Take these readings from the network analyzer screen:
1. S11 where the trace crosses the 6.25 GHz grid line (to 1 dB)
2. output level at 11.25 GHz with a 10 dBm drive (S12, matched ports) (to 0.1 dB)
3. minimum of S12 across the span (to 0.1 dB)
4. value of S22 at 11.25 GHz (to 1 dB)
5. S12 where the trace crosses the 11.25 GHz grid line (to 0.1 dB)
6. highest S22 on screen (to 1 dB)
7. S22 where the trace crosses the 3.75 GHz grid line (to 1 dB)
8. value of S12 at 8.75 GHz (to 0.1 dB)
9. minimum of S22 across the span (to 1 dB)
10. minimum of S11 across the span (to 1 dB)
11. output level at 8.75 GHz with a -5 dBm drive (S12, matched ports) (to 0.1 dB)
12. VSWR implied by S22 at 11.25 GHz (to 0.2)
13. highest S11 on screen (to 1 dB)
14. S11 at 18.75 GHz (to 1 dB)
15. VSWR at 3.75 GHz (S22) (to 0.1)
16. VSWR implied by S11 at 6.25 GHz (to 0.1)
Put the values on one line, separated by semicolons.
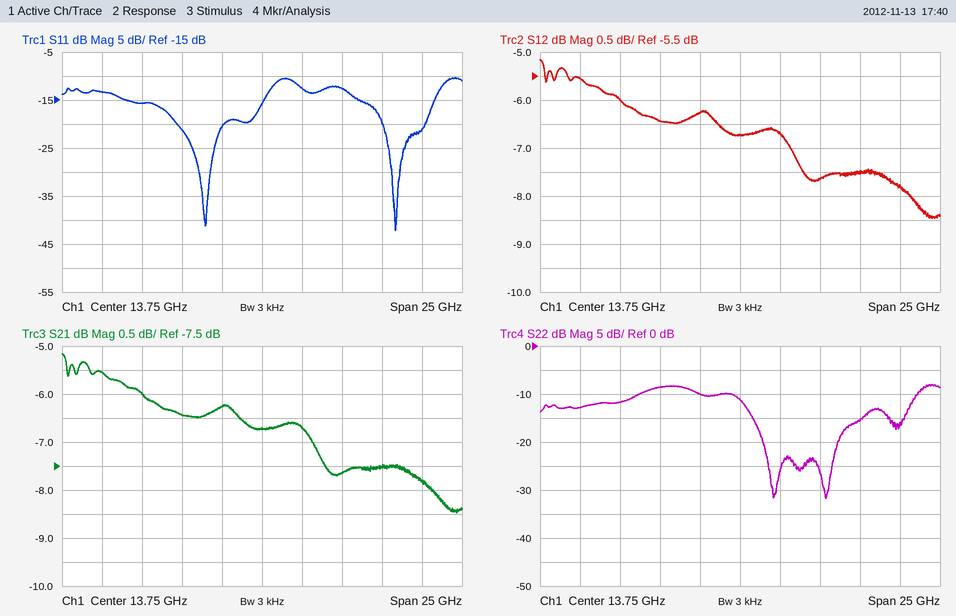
-16 dB; 3.7 dBm; -8.5 dB; -10 dB; -6.3 dB; -8 dB; -13 dB; -6.4 dB; -32 dB; -42 dB; -11.4 dBm; 2.0; -10 dB; -13 dB; 1.6; 1.4
